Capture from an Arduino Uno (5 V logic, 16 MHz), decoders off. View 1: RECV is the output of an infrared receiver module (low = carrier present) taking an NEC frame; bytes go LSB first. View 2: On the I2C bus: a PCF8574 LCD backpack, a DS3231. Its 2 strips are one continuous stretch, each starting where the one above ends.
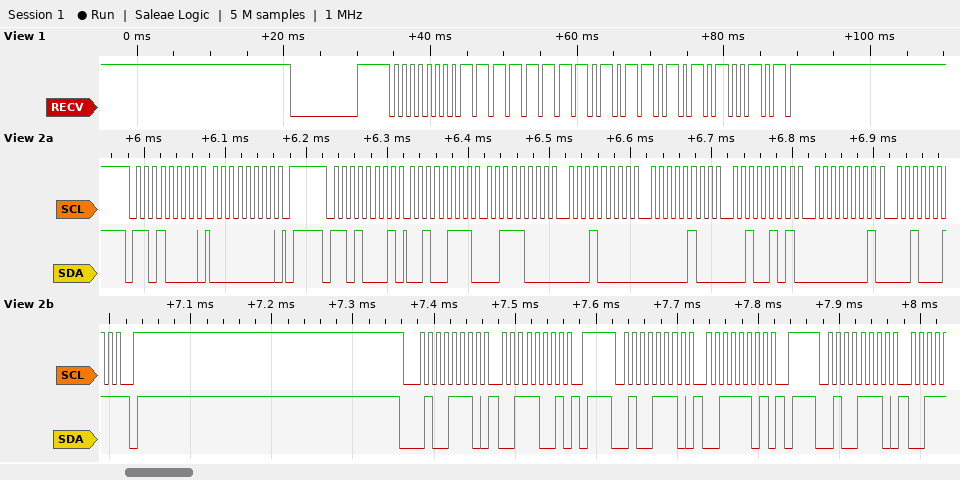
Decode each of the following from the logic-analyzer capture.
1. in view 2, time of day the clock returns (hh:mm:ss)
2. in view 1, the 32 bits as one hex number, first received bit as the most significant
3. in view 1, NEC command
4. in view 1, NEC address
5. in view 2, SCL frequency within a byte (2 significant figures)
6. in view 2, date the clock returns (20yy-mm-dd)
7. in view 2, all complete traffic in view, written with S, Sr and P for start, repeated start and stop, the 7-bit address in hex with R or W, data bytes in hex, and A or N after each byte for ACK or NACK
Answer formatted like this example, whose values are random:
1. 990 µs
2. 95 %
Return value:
1. 10:38:27
2. 0x00FF5AA5
3. 0x5A
4. 0x00
5. 100 kHz
6. 2023-01-25
7. S 68W A 00 A P S 68R A 27 A 38 A 10 A 04 A 25 A 01 A 23 N P S 27W A 39 A P S 27W A 3D A P S 27W A
